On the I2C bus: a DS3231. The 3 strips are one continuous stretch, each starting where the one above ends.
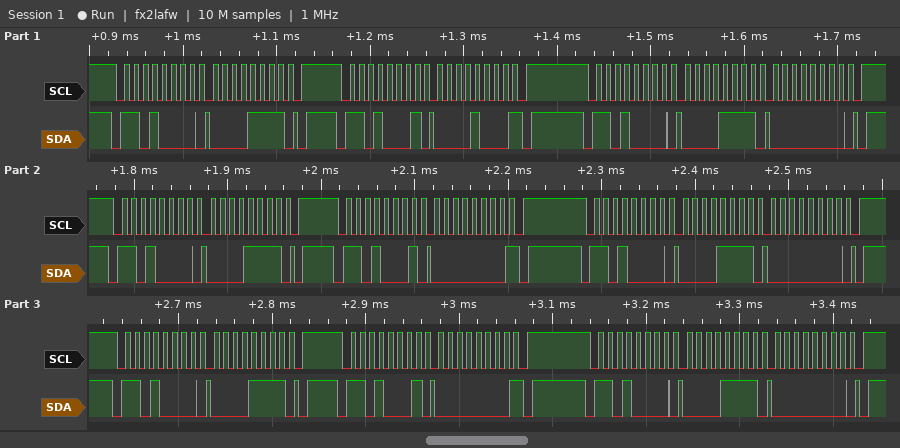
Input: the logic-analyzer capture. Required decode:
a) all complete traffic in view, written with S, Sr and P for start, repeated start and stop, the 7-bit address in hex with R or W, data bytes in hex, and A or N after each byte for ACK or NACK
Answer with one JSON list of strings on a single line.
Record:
["S 68W A 0F A P S 68R A 08 N P S 68W A 0F A 00 A P S 68W A 0F A P S 68R A 00 N P S 68W A 0F A 00 A P S 68W A 0F A P S 68R A 00 N P S 68W A 0F A 00 A P"]
